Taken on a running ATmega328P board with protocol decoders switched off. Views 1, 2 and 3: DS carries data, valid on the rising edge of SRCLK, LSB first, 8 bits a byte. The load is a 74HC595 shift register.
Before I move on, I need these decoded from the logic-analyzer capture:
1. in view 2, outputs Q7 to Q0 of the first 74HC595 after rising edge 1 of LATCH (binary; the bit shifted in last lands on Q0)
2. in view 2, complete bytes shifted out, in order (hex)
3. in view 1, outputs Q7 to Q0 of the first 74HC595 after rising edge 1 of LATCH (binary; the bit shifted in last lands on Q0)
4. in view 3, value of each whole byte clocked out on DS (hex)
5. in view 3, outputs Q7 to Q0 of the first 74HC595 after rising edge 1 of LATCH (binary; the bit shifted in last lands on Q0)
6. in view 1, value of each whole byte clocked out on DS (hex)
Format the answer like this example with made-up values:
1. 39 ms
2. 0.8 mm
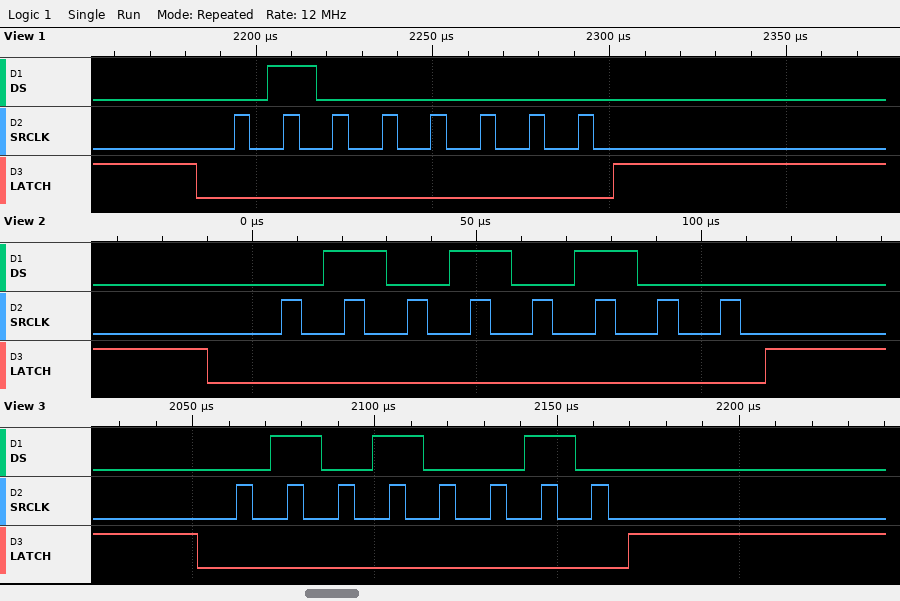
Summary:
1. 01010100
2. 2A
3. 01000000
4. 4A
5. 01010010
6. 02
